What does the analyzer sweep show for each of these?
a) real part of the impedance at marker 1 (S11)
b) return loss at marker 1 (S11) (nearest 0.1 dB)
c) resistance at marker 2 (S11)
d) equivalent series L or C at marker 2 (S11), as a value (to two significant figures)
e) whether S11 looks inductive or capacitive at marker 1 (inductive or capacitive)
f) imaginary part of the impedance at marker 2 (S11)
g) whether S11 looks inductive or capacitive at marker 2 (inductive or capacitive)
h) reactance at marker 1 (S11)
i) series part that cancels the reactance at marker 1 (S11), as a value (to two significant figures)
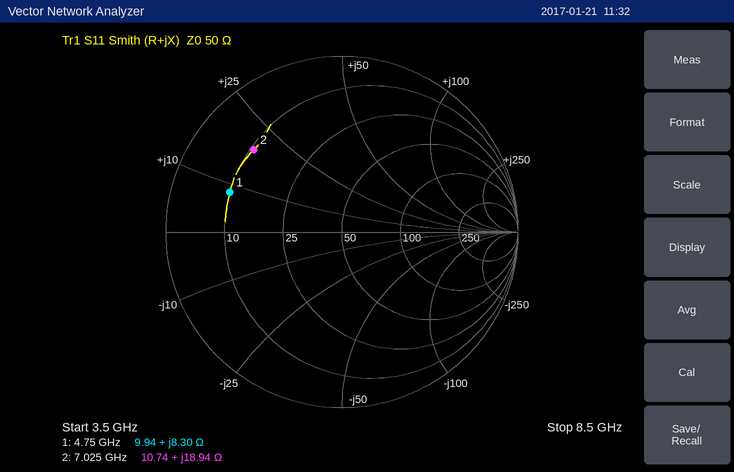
9.94 Ω
3.4 dB
10.74 Ω
430 pH
inductive
+18.94 Ω
inductive
+8.30 Ω
4.0 pF
